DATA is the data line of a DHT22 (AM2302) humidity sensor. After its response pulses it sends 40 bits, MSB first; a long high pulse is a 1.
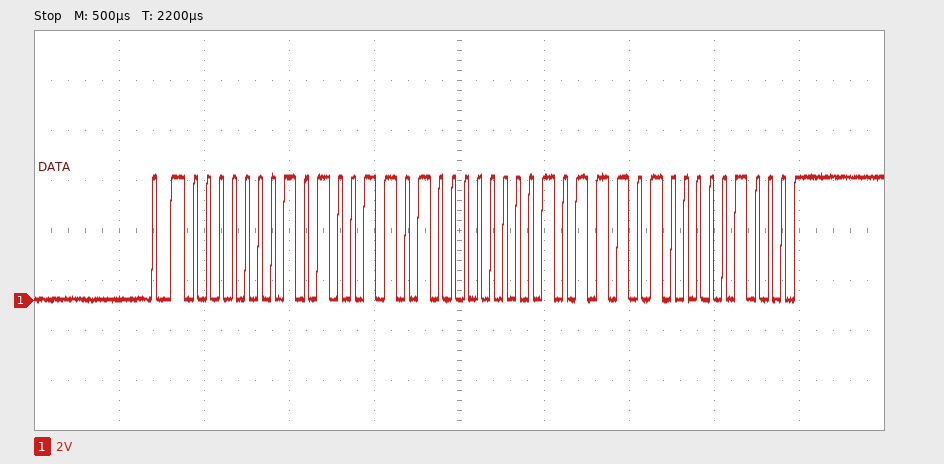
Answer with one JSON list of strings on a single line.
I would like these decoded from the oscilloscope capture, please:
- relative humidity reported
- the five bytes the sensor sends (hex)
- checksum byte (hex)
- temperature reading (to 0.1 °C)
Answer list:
["33.3 %", "01 4D 00 BA 08", "0x08", "18.6 °C"]
